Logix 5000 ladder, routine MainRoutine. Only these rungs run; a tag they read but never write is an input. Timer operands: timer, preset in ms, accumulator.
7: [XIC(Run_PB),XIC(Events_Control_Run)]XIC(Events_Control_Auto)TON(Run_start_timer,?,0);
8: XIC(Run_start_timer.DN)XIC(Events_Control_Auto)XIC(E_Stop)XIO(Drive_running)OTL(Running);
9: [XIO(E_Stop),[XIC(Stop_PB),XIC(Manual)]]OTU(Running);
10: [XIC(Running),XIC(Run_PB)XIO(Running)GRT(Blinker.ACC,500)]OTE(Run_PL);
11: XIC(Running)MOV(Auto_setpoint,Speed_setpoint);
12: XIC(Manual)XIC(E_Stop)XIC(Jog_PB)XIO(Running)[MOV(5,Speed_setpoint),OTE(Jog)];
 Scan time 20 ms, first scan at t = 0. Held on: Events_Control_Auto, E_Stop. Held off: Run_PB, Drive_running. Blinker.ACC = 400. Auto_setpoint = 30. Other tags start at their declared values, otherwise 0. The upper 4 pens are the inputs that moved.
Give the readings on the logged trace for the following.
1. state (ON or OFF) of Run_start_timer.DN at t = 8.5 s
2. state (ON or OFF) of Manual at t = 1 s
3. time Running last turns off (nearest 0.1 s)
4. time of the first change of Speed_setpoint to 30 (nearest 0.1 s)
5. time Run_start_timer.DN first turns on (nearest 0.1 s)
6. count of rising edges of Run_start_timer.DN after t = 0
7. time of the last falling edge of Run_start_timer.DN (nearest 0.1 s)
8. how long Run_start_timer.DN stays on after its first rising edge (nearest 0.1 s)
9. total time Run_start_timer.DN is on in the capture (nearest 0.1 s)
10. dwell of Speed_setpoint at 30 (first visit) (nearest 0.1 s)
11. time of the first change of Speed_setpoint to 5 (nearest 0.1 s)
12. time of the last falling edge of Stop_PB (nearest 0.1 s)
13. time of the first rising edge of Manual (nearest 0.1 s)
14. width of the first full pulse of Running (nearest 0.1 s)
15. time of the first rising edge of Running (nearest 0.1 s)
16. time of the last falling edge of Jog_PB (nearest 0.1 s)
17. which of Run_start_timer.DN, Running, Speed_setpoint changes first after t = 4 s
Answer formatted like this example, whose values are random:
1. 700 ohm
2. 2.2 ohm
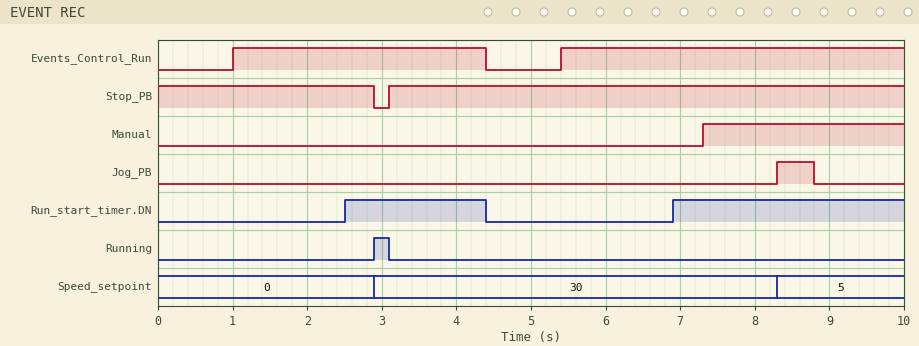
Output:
1. ON
2. OFF
3. 3.1 s
4. 2.9 s
5. 2.5 s
6. 2
7. 4.4 s
8. 1.9 s
9. 5.0 s
10. 5.4 s
11. 8.3 s
12. 2.9 s
13. 7.3 s
14. 0.2 s
15. 2.9 s
16. 8.8 s
17. Run_start_timer.DN
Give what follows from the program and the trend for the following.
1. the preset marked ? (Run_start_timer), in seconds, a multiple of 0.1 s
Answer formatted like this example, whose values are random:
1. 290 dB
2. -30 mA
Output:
1. 1.5 s
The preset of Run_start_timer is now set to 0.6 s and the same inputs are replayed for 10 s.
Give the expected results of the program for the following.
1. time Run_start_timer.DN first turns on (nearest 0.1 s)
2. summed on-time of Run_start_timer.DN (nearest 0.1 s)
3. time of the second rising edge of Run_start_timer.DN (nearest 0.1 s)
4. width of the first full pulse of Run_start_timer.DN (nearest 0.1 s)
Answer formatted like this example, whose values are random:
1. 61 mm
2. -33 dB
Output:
1. 1.6 s
2. 6.8 s
3. 6.0 s
4. 2.8 s
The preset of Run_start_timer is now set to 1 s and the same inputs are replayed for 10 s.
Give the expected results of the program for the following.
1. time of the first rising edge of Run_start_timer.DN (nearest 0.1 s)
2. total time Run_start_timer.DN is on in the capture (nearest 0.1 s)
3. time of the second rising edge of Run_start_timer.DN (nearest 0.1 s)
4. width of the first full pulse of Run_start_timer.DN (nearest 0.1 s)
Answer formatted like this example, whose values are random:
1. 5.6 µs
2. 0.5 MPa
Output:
1. 2.0 s
2. 6.0 s
3. 6.4 s
4. 2.4 s
